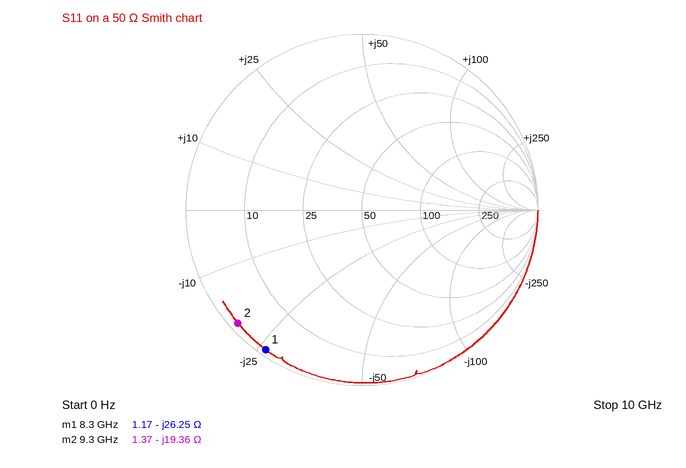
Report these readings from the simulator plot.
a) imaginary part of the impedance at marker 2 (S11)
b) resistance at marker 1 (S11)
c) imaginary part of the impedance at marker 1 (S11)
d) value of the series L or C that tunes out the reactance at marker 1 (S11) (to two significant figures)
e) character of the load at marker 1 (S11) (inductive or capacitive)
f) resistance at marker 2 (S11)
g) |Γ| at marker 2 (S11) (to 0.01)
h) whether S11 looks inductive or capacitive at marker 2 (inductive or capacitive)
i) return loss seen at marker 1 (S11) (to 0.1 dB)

-19.36 Ω
1.17 Ω
-26.25 Ω
500 pH
capacitive
1.37 Ω
0.95
capacitive
0.3 dB
